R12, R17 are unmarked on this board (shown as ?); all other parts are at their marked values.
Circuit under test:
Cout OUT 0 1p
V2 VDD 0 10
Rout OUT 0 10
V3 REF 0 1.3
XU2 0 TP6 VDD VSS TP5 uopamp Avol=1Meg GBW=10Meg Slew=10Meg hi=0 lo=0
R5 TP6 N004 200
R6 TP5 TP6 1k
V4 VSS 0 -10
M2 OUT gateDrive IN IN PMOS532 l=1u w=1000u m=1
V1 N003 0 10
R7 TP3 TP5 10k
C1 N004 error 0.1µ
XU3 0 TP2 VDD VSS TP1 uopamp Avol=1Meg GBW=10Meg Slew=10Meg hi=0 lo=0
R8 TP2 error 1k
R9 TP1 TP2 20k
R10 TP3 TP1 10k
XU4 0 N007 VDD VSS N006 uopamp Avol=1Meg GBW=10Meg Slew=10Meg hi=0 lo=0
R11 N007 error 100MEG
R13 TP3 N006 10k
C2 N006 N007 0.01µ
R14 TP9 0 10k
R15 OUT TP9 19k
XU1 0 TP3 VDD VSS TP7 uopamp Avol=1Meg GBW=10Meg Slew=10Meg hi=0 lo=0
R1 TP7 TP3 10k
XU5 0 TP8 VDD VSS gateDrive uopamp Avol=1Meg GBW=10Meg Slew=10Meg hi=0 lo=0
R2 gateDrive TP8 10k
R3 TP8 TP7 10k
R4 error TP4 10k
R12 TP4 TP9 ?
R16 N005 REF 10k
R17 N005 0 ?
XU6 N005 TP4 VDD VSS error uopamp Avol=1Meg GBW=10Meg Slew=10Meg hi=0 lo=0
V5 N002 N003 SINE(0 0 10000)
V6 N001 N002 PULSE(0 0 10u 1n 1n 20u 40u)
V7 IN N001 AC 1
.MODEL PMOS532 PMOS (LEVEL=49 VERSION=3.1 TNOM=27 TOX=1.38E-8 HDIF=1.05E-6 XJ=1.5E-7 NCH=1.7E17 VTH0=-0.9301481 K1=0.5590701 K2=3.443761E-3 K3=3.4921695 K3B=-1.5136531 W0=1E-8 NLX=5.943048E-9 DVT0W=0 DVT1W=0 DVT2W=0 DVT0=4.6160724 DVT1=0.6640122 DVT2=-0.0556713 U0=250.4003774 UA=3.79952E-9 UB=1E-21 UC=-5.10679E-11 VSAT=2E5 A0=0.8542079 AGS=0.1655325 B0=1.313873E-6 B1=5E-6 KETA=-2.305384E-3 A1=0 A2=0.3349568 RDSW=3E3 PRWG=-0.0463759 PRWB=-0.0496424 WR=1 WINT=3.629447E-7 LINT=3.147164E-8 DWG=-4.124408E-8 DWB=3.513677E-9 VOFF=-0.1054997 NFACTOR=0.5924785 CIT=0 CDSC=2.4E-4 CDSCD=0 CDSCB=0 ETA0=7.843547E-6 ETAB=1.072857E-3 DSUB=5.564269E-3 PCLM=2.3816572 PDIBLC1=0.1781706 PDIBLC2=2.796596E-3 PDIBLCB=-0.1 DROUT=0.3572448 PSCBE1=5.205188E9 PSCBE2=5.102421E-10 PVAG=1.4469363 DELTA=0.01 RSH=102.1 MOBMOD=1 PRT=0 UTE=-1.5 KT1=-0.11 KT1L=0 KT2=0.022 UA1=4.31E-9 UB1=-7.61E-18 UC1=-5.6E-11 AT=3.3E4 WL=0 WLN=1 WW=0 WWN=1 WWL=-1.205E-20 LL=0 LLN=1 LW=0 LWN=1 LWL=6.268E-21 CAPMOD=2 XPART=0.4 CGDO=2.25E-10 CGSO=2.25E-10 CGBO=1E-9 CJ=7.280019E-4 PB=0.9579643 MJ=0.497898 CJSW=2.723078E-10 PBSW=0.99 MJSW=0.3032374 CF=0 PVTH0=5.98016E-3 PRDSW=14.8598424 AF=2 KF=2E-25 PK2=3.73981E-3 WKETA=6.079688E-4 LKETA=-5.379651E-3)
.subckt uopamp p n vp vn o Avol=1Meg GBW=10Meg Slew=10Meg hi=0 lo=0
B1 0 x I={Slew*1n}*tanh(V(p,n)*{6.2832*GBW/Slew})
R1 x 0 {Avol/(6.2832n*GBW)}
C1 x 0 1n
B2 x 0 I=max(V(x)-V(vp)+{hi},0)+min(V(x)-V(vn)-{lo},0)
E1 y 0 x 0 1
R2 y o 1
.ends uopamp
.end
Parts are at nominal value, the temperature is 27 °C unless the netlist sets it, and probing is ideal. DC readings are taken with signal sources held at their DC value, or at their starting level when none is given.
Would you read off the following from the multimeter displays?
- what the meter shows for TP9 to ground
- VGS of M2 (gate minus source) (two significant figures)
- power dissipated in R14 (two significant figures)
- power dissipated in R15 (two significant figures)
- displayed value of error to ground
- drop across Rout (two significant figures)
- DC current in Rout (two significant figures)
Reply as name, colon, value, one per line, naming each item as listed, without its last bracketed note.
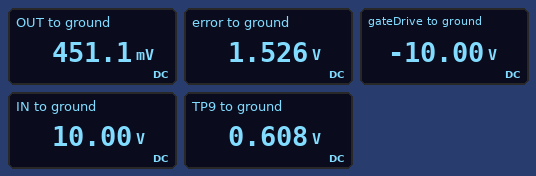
what the meter shows for TP9 to ground: 0.608 V
VGS of M2 (gate minus source): -20 V
power dissipated in R14: 37 µW
power dissipated in R15: 1.3 µW
displayed value of error to ground: 1.526 V
drop across Rout: 450 mV
DC current in Rout: 45 mA
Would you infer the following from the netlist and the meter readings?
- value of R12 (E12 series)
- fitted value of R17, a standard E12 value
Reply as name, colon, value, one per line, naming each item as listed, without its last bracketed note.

value of R12: 3.3 kΩ
fitted value of R17, a standard E12 value: 18 kΩ
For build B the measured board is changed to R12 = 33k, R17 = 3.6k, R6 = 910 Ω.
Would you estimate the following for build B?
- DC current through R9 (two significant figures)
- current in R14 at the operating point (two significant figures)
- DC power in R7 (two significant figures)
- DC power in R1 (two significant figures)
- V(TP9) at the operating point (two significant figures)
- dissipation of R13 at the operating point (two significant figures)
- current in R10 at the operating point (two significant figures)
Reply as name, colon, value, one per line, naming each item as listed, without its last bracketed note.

DC current through R9: 390 µA
current in R14 at the operating point: 19 µA
DC power in R7: 380 µW
DC power in R1: 14 mW
V(TP9) at the operating point: 190 mV
dissipation of R13 at the operating point: 6.5 mW
current in R10 at the operating point: 590 µA
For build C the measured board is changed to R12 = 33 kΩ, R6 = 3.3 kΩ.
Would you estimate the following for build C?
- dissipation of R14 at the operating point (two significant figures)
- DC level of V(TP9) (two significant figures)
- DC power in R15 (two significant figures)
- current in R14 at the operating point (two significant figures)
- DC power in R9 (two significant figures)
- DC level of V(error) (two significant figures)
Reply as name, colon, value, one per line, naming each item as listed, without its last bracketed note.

dissipation of R14 at the operating point: 7.2 µW
DC level of V(TP9): 270 mV
DC power in R15: 1.8 µW
current in R14 at the operating point: 27 µA
DC power in R9: 5.5 mW
DC level of V(error): 1.0 V
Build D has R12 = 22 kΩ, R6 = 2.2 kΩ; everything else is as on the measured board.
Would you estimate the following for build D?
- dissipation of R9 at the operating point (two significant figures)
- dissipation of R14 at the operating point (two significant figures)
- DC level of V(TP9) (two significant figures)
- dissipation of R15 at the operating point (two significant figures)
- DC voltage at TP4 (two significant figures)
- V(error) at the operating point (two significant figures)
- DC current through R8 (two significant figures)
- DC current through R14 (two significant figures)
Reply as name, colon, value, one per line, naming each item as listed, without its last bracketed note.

dissipation of R9 at the operating point: 5.6 mW
dissipation of R14 at the operating point: 9.7 µW
DC level of V(TP9): 310 mV
dissipation of R15 at the operating point: 1.0 µW
DC voltage at TP4: 840 mV
V(error) at the operating point: 1.1 V
DC current through R8: 530 µA
DC current through R14: 31 µA
